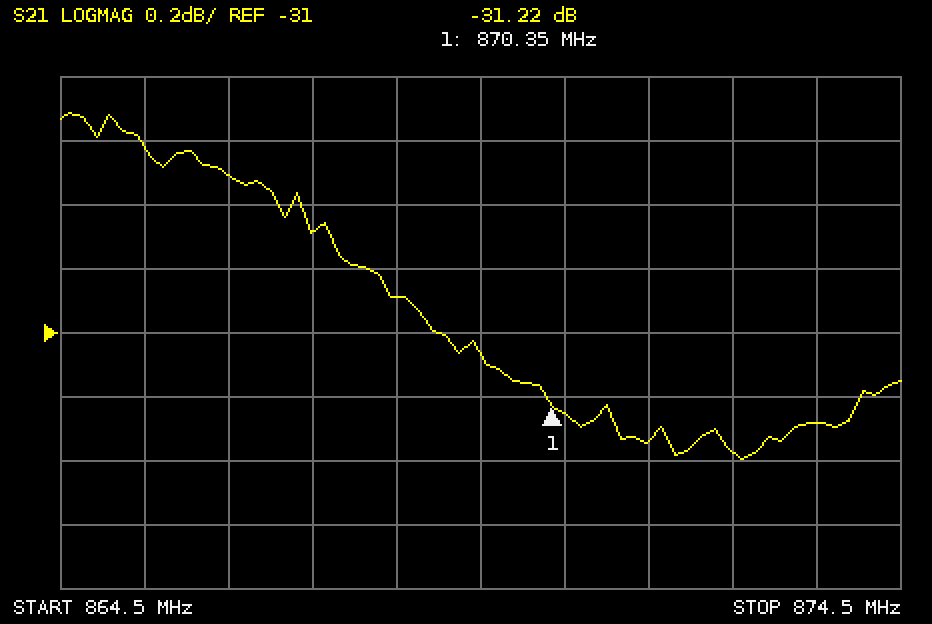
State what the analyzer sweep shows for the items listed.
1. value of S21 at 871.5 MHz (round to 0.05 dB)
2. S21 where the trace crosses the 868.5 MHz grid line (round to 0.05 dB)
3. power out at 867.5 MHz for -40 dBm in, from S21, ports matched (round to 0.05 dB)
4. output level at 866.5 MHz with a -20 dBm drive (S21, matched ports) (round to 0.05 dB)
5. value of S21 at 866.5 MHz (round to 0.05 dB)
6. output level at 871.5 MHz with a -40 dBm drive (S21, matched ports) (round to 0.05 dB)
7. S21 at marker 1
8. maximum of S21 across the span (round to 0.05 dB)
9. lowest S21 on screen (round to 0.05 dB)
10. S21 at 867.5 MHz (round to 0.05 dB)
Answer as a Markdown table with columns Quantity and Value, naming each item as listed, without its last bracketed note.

| Quantity | Value |
|---|---|
| value of S21 at 871.5 MHz | -31.35 dB |
| S21 where the trace crosses the 868.5 MHz grid line | -30.90 dB |
| power out at 867.5 MHz for -40 dBm in, from S21, ports matched | -70.70 dBm |
| output level at 866.5 MHz with a -20 dBm drive (S21, matched ports) | -50.50 dBm |
| value of S21 at 866.5 MHz | -30.50 dB |
| output level at 871.5 MHz with a -40 dBm drive (S21, matched ports) | -71.35 dBm |
| S21 at marker 1 | -31.22 dB |
| maximum of S21 across the span | -30.30 dB |
| lowest S21 on screen | -31.40 dB |
| S21 at 867.5 MHz | -30.70 dB |
